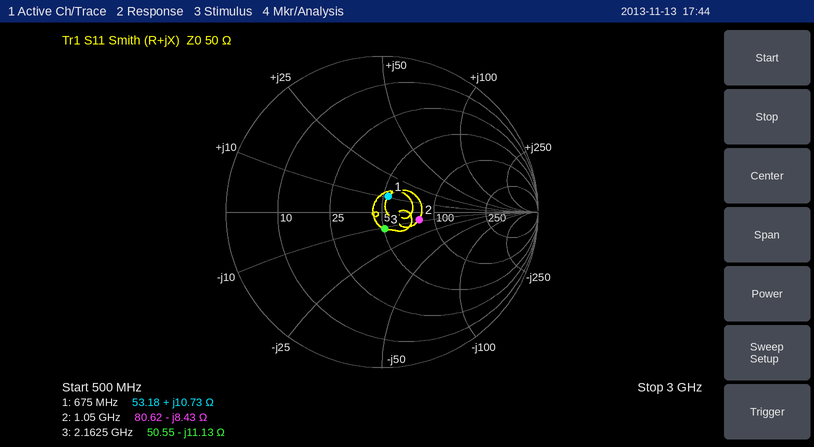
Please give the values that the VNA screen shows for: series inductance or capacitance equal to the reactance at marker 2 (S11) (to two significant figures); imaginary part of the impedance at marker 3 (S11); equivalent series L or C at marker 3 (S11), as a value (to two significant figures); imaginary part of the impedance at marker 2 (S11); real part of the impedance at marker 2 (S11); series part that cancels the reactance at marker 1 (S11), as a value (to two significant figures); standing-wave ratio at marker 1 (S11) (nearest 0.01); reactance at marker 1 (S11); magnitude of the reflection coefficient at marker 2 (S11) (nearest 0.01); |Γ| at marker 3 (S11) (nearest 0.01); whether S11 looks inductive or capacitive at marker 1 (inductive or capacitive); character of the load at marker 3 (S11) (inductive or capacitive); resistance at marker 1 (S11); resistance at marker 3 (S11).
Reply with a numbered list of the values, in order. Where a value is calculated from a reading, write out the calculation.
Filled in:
1. C = 1/(2π × 1.05 GHz × 8.43 Ω) ≈ 18 pF
2. -11.13 Ω
3. C = 1/(2π × 2.1625 GHz × 11.13 Ω) ≈ 6.6 pF
4. -8.43 Ω
5. 80.62 Ω
6. C = 1/(2π × 675 MHz × 10.73 Ω) ≈ 22 pF
7. 1.24
8. +10.73 Ω
9. 0.24
10. 0.11
11. inductive
12. capacitive
13. 53.18 Ω
14. 50.55 Ω
